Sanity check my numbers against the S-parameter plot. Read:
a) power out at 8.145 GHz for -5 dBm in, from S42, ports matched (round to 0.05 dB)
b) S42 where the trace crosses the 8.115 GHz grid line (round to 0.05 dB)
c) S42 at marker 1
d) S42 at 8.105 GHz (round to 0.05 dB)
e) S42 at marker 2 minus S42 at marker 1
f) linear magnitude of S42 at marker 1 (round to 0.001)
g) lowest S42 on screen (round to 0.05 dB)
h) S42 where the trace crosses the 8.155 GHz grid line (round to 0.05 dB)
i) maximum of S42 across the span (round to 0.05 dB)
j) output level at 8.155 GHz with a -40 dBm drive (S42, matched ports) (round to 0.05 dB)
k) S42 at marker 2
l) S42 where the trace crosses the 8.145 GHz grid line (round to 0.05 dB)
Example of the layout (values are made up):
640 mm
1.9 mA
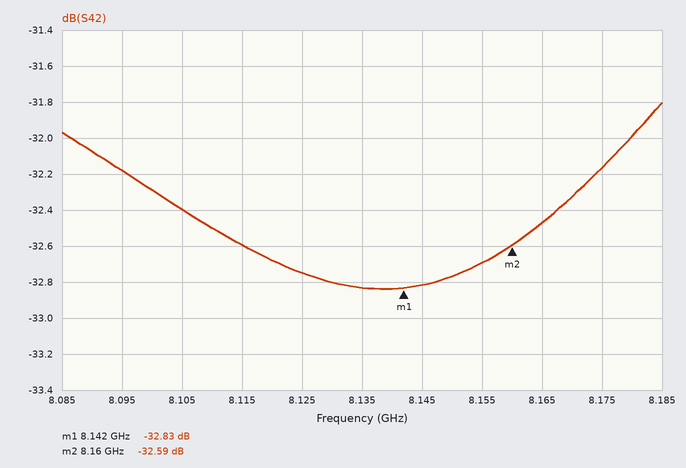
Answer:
-37.80 dBm
-32.60 dB
-32.83 dB
-32.40 dB
0.24 dB
0.023
-32.85 dB
-32.70 dB
-31.80 dB
-72.70 dBm
-32.59 dB
-32.80 dB
